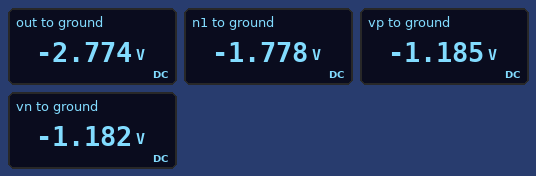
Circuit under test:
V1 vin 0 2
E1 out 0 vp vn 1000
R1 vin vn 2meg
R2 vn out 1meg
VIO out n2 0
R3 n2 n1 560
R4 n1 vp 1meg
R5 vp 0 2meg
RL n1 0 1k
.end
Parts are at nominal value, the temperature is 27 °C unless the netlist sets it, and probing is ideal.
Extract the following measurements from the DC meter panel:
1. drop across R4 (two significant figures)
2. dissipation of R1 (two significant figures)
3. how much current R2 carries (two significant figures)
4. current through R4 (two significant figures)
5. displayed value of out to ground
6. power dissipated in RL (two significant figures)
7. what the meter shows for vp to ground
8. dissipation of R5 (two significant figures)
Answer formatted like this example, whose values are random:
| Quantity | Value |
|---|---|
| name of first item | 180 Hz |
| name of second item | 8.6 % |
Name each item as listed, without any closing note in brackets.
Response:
| Quantity | Value |
|---|---|
| drop across R4 | 590 mV |
| dissipation of R1 | 5.1 µW |
| how much current R2 carries | 1.6 µA |
| current through R4 | 590 nA |
| displayed value of out to ground | -2.774 V |
| power dissipated in RL | 3.2 mW |
| what the meter shows for vp to ground | -1.185 V |
| dissipation of R5 | 700 nW |
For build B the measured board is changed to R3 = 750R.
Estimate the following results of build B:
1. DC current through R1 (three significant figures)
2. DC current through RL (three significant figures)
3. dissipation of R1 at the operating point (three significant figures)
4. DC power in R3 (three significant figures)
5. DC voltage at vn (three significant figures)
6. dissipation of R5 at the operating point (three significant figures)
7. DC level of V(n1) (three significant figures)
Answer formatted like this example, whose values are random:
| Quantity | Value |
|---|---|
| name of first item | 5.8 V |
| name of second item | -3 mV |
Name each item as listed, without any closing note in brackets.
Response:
| Quantity | Value |
|---|---|
| DC current through R1 | 1.44 µA |
| DC current through RL | 1.33 mA |
| dissipation of R1 at the operating point | 4.16 µW |
| DC power in R3 | 1.32 mW |
| DC voltage at vn | -883 mV |
| dissipation of R5 at the operating point | 392 nW |
| DC level of V(n1) | -1.33 V |
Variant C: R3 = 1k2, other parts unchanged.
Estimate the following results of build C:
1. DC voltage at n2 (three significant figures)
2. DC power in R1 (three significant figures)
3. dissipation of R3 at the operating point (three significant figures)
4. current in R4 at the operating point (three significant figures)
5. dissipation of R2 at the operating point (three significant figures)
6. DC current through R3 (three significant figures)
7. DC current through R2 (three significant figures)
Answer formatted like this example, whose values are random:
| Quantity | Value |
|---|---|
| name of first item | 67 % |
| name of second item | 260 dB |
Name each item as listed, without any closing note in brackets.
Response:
| Quantity | Value |
|---|---|
| DC voltage at n2 | -1.83 V |
| DC power in R1 | 3.26 µW |
| dissipation of R3 at the operating point | 829 µW |
| current in R4 at the operating point | 277 nA |
| dissipation of R2 at the operating point | 1.63 µW |
| DC current through R3 | 831 µA |
| DC current through R2 | 1.28 µA |
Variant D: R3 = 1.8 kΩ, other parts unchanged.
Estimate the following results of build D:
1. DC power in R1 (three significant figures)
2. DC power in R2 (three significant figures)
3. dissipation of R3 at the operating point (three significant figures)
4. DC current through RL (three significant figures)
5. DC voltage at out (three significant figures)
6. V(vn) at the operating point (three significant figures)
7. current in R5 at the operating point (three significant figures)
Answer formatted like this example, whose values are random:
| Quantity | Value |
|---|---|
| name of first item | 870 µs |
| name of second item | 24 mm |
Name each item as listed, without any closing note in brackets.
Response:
| Quantity | Value |
|---|---|
| DC power in R1 | 2.80 µW |
| DC power in R2 | 1.40 µW |
| dissipation of R3 at the operating point | 553 µW |
| DC current through RL | 554 µA |
| DC voltage at out | -1.55 V |
| V(vn) at the operating point | -368 mV |
| current in R5 at the operating point | 185 nA |
